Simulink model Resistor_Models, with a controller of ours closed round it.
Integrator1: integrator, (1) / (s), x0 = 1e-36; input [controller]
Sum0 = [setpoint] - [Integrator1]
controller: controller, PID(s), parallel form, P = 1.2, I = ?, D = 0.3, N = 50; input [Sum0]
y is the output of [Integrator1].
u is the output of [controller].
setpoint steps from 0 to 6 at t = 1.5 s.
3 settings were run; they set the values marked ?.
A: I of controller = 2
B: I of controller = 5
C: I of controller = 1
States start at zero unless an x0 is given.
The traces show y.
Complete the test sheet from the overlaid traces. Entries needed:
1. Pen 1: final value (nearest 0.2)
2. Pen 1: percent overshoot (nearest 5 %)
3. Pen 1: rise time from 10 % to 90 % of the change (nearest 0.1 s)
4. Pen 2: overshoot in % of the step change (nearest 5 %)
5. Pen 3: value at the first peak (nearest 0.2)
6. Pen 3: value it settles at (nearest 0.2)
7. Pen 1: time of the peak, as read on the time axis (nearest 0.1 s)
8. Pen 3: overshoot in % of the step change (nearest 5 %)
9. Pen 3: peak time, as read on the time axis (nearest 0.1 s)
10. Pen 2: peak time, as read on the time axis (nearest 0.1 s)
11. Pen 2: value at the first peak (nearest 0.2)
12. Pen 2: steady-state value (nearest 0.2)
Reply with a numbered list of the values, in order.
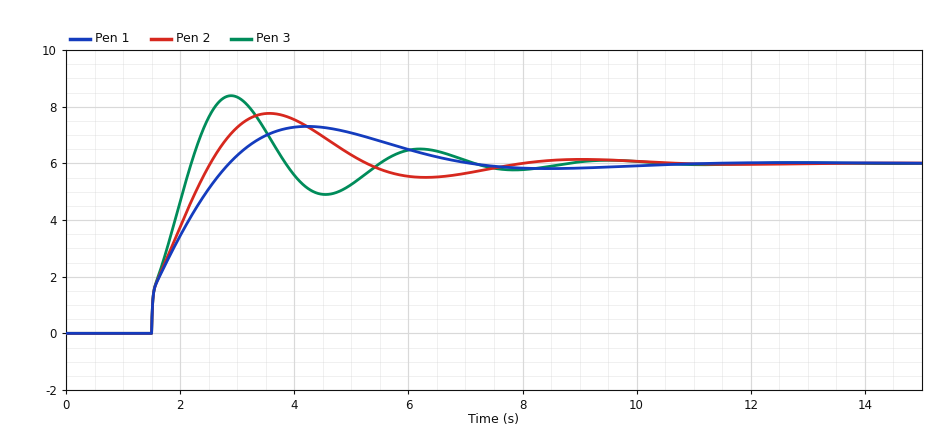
1. 6.0
2. 20 %
3. 1.1 s
4. 30 %
5. 8.4
6. 6.0
7. 4.2 s
8. 40 %
9. 2.9 s
10. 3.6 s
11. 7.8
12. 6.0
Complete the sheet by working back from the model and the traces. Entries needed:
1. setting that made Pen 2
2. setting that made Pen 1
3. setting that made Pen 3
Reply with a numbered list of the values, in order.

1. A
2. C
3. B
